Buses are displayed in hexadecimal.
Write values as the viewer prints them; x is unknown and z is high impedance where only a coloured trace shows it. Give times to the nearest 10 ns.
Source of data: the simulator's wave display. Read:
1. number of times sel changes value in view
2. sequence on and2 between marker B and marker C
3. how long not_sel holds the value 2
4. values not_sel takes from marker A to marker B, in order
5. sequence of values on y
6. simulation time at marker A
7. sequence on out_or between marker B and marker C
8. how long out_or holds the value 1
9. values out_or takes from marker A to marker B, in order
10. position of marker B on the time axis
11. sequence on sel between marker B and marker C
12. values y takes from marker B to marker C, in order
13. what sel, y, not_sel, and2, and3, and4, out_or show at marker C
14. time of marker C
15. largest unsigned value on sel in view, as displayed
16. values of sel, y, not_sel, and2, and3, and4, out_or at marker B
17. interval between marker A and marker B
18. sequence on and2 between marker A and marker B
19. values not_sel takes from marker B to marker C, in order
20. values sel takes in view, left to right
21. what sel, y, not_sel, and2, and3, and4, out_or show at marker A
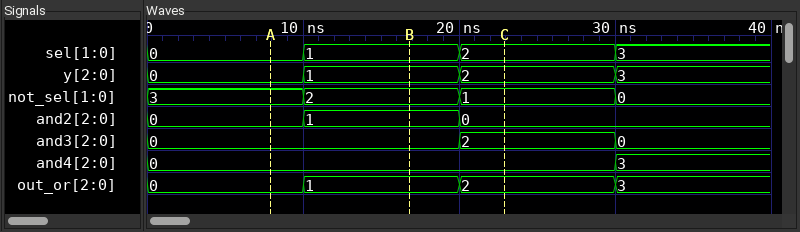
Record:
3
1, 0
10 ns
3, 2
0, 1, 2, 3
10 ns
1, 2
10 ns
0, 1
20 ns
1, 2
1, 2
sel=2, y=2, not_sel=1, and2=0, and3=2, and4=0, out_or=2
20 ns
3
sel=1, y=1, not_sel=2, and2=1, and3=0, and4=0, out_or=1
10 ns
0, 1
2, 1
0, 1, 2, 3
sel=0, y=0, not_sel=3, and2=0, and3=0, and4=0, out_or=0
